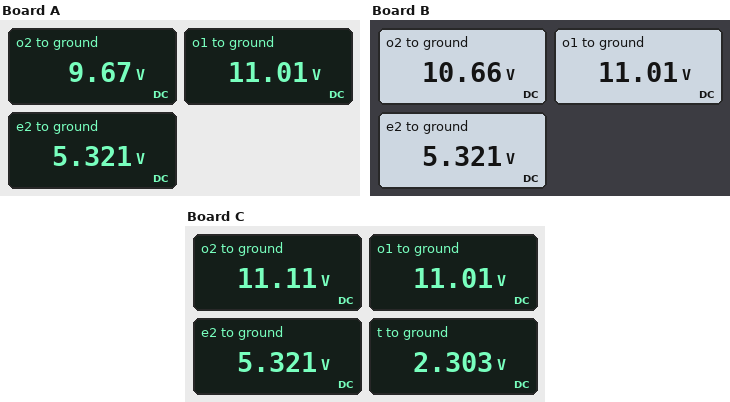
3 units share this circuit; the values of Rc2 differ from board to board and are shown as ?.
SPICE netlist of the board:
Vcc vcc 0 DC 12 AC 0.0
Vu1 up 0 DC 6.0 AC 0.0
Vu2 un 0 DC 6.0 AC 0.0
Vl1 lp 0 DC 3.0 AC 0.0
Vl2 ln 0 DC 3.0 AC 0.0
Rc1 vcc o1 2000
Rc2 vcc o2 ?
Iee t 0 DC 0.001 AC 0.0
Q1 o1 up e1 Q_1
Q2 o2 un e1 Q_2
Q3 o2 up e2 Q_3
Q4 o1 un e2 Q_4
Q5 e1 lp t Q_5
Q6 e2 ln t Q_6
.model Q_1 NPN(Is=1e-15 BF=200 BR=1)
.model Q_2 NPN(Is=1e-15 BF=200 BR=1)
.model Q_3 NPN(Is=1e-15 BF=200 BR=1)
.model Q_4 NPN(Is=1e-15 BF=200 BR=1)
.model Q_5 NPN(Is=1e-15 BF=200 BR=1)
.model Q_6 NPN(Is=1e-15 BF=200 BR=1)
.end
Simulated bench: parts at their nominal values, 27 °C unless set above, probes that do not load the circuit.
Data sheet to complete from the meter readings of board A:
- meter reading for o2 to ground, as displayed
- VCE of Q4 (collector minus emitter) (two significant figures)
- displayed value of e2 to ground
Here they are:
9.67 V
5.7 V
5.321 V
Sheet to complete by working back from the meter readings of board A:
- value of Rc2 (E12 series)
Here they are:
4.7 kΩ
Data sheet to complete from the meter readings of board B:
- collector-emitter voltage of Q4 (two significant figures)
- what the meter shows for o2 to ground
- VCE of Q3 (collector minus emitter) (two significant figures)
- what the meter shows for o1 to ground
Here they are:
5.7 V
10.66 V
5.3 V
11.01 V
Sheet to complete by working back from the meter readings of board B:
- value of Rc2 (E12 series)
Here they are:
2.7 kΩ
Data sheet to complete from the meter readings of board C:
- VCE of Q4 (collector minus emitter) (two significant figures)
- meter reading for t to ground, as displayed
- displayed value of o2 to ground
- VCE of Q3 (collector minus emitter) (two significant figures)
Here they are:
5.7 V
2.303 V
11.11 V
5.8 V
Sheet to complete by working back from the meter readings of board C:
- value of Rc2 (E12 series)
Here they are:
1.8 kΩ
